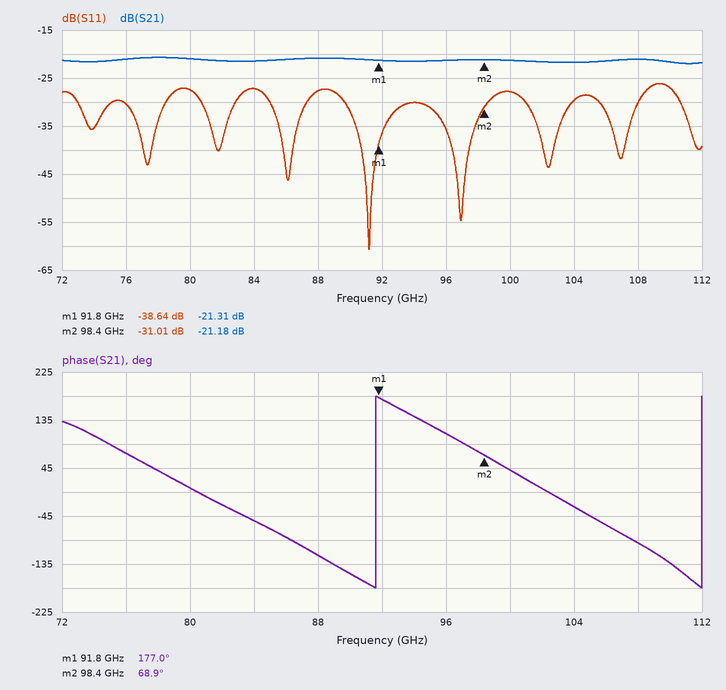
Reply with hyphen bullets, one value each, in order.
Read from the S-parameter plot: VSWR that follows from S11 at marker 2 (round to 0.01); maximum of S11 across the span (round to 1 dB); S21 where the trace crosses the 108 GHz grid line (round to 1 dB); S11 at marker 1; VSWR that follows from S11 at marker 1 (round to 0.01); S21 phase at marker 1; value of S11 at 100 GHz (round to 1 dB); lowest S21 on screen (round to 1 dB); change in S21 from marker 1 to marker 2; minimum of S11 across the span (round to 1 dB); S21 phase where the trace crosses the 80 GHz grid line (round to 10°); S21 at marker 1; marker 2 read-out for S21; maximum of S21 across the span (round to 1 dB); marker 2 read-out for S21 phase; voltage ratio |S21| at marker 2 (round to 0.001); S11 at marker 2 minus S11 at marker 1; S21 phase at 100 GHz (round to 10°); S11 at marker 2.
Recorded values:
- 1.06
- -26 dB
- -21 dB
- -38.64 dB
- 1.02
- 177.0°
- -28 dB
- -22 dB
- 0.13 dB
- -61 dB
- 10°
- -21.31 dB
- -21.18 dB
- -21 dB
- 68.9°
- 0.087
- 7.63 dB
- 40°
- -31.01 dB
